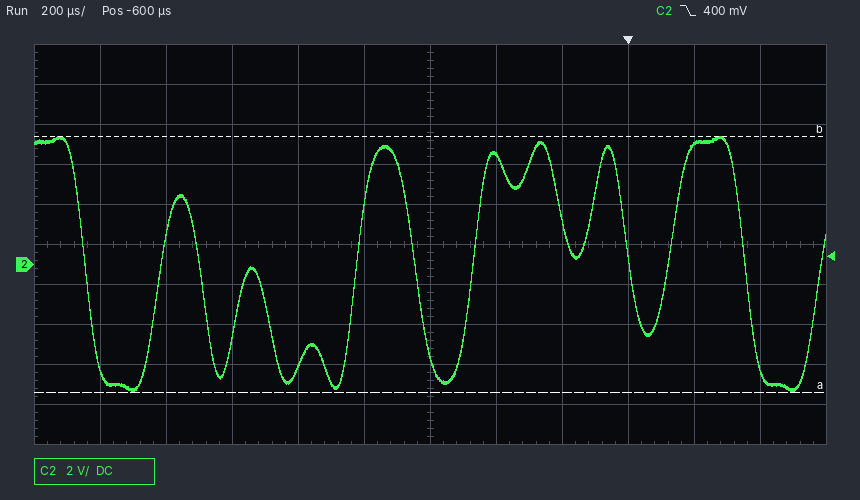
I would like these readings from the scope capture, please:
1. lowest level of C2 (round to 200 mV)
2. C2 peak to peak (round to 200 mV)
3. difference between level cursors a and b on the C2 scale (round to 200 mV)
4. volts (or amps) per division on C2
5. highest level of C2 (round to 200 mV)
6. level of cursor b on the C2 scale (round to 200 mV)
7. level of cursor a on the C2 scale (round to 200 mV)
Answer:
-6.4 V
12.8 V
12.8 V
2 V
6.4 V
6.4 V
-6.4 V
